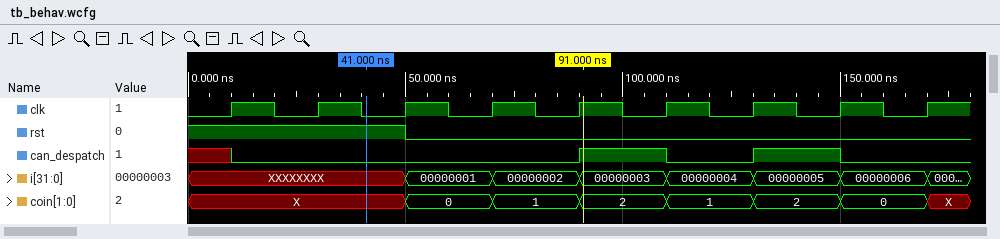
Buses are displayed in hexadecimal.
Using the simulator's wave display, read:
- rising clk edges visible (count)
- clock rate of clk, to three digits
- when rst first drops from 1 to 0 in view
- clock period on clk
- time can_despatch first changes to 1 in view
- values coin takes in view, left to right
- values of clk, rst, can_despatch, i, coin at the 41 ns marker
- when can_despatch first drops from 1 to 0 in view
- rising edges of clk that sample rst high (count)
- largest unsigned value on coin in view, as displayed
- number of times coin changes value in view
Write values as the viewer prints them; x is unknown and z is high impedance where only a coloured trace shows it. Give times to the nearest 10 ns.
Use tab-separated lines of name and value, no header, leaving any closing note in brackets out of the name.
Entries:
rising clk edges visible	9
clock rate of clk, to three digits	50.0 MHz
when rst first drops from 1 to 0 in view	50 ns
clock period on clk	20 ns
time can_despatch first changes to 1 in view	90 ns
values coin takes in view, left to right	X, 0, 1, 2, 1, 2, 0, X
values of clk, rst, can_despatch, i, coin at the 41 ns marker	clk=0, rst=1, can_despatch=0, i=XXXXXXXX, coin=X
when can_despatch first drops from 1 to 0 in view	110 ns
rising edges of clk that sample rst high	3
largest unsigned value on coin in view, as displayed	2
number of times coin changes value in view	7
